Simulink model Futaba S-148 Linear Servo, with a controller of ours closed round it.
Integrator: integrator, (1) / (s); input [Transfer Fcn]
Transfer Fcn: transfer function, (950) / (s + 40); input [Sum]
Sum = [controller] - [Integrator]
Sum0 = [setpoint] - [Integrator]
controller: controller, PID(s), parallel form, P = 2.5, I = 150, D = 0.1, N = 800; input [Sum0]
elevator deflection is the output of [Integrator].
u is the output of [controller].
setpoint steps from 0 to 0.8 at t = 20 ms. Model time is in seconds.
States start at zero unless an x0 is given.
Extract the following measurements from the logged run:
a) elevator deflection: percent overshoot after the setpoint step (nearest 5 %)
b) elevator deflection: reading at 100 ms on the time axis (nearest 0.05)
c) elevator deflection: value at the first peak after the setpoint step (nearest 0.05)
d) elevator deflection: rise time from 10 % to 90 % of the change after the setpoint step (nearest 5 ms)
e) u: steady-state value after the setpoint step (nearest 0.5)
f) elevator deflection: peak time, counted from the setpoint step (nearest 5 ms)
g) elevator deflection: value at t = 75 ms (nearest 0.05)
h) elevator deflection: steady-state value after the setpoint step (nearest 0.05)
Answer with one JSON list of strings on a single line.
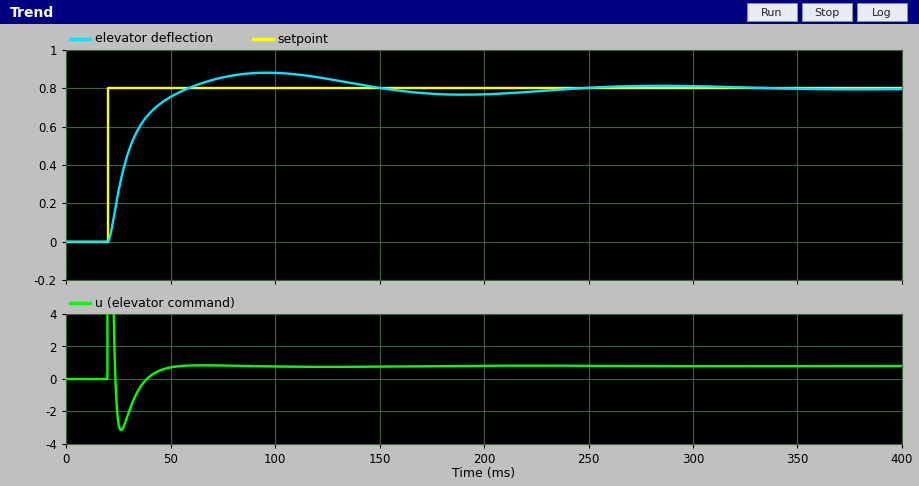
["10 %", "0.90", "0.90", "25 ms", "1.0", "75 ms", "0.85", "0.80"]
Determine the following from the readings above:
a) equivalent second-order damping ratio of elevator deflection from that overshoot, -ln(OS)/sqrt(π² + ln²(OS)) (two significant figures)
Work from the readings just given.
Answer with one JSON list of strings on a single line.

["0.59"]
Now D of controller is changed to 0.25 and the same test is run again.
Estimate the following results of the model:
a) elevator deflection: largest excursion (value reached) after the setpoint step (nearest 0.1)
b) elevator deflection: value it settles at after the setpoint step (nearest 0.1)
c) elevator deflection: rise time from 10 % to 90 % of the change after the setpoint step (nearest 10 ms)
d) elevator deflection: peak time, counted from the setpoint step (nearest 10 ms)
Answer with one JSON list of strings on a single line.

["0.8", "0.8", "30 ms", "150 ms"]
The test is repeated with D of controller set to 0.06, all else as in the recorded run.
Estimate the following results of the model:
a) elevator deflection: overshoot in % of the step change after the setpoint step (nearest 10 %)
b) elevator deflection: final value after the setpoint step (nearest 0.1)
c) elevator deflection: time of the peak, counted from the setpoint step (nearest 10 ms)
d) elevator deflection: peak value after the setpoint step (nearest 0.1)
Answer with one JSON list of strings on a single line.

["20 %", "0.8", "60 ms", "1.0"]
